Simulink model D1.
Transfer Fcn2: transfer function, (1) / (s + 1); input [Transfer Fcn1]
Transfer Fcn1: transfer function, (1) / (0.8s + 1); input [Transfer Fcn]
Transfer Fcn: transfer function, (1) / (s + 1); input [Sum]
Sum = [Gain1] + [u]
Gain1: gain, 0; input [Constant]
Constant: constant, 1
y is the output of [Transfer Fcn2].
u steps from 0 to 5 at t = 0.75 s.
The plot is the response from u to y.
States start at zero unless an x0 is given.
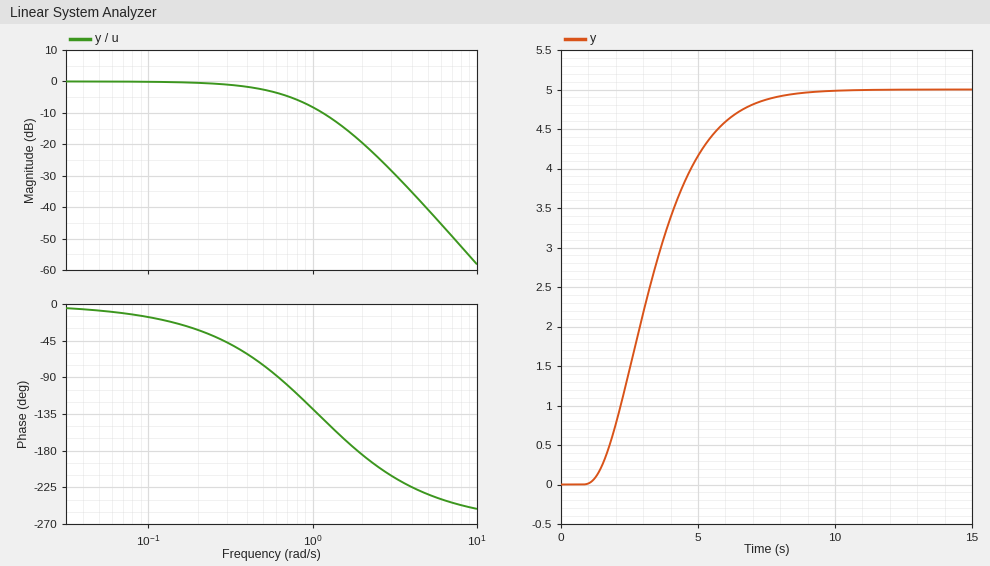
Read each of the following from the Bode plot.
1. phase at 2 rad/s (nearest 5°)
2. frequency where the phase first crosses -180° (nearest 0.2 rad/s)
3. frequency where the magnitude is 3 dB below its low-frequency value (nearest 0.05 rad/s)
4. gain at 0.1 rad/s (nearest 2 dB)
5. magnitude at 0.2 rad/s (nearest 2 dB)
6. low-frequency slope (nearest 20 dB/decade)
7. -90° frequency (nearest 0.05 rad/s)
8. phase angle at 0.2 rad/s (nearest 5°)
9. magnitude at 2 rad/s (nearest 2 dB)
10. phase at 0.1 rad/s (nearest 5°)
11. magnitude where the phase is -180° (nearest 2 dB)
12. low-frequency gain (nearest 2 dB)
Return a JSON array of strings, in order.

["-185°", "1.8 rad/s", "0.55 rad/s", "0 dB", "0 dB", "0 dB/decade", "0.60 rad/s", "-30°", "-20 dB", "-15°", "-18 dB", "0 dB"]
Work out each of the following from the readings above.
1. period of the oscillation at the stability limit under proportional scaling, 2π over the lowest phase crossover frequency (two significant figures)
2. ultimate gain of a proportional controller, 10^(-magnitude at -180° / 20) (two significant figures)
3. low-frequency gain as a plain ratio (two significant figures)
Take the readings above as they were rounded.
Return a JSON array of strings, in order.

["3.5 s", "7.9", "1.0"]
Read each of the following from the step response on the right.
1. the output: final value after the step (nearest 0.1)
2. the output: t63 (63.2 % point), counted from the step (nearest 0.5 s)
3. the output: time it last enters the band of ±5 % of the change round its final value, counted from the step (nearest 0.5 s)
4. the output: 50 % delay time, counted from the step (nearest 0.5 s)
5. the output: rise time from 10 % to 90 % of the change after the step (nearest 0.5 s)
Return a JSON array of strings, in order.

["5.0", "3.0 s", "6.0 s", "2.5 s", "4.0 s"]
